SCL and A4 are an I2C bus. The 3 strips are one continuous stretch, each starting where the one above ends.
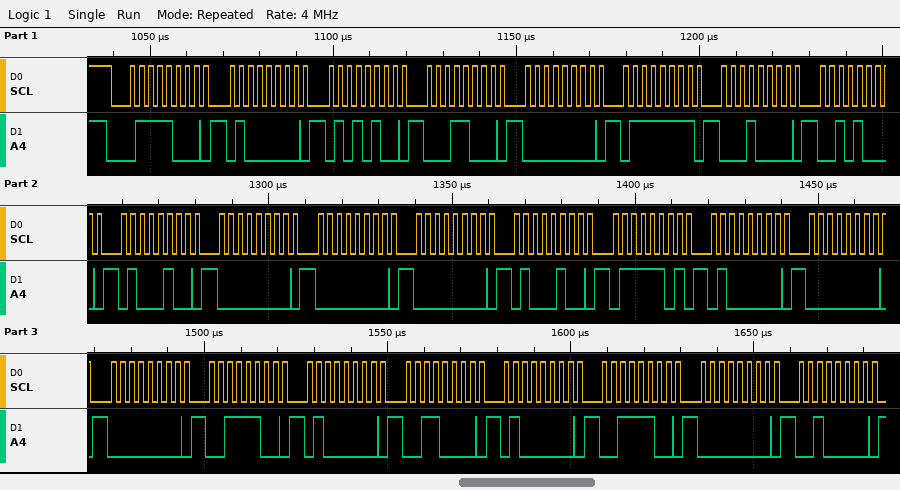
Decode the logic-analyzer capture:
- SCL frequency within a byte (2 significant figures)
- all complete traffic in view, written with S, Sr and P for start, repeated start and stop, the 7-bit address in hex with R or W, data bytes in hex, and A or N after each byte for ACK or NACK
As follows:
400 kHz
S 3CW A 40 A 54 A 18 A 00 A 7F A 10 A 28 A 44 A 00 A 00 A 00 A 44 A 7D A 40 A 00 A 00 A 3C A 40 A 30 A 40 A 3C A 00 A 20 A
